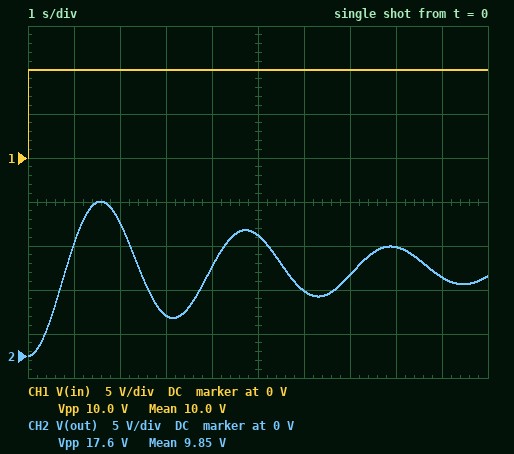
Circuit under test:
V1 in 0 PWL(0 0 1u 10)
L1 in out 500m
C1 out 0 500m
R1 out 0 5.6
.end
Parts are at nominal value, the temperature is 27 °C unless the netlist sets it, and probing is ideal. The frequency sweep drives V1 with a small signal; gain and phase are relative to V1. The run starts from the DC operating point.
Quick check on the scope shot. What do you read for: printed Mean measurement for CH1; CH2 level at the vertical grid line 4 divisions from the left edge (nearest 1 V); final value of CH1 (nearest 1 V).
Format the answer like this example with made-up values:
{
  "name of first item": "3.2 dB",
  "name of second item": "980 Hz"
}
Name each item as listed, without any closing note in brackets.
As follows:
{
  "printed Mean measurement for CH1": "10.0 V",
  "CH2 level at the vertical grid line 4 divisions from the left edge": "10 V",
  "final value of CH1": "10 V"
}
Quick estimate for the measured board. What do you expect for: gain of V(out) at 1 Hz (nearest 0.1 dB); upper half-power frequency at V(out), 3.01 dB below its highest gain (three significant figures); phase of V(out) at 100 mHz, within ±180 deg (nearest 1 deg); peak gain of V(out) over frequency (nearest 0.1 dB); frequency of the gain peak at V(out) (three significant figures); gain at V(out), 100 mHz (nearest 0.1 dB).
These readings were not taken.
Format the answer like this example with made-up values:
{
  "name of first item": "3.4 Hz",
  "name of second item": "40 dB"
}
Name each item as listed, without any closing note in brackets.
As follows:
{
  "gain of V(out) at 1 Hz": "-19.0 dB",
  "upper half-power frequency at V(out), 3.01 dB below its highest gain": "343 mHz",
  "phase of V(out) at 100 mHz, within ±180 deg": "-4 deg",
  "peak gain of V(out) over frequency": "15.0 dB",
  "frequency of the gain peak at V(out)": "316 mHz",
  "gain at V(out), 100 mHz": "0.9 dB"
}
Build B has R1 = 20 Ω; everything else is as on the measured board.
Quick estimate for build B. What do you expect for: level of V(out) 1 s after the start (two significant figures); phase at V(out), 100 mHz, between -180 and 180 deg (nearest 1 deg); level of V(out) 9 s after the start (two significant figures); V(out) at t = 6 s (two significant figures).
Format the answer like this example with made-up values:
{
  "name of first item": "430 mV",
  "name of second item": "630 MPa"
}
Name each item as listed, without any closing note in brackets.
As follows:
{
  "level of V(out) 1 s after the start": "14 V",
  "phase at V(out), 100 mHz, between -180 and 180 deg": "-1 deg",
  "level of V(out) 9 s after the start": "5.9 V",
  "V(out) at t = 6 s": "3.9 V"
}
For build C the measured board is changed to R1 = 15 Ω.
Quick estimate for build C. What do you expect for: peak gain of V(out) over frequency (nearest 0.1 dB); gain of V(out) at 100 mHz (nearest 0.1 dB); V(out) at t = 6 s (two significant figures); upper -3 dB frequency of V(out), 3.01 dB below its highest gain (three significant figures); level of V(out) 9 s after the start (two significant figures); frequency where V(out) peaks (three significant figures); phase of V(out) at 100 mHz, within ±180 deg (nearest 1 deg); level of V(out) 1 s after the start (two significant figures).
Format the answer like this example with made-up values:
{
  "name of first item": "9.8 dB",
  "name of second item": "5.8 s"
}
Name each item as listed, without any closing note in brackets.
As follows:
{
  "peak gain of V(out) over frequency": "23.5 dB",
  "gain of V(out) at 100 mHz": "0.9 dB",
  "V(out) at t = 6 s": "4.5 V",
  "upper -3 dB frequency of V(out), 3.01 dB below its highest gain": "328 mHz",
  "level of V(out) 9 s after the start": "6.6 V",
  "frequency where V(out) peaks": "318 mHz",
  "phase of V(out) at 100 mHz, within ±180 deg": "-1 deg",
  "level of V(out) 1 s after the start": "14 V"
}
